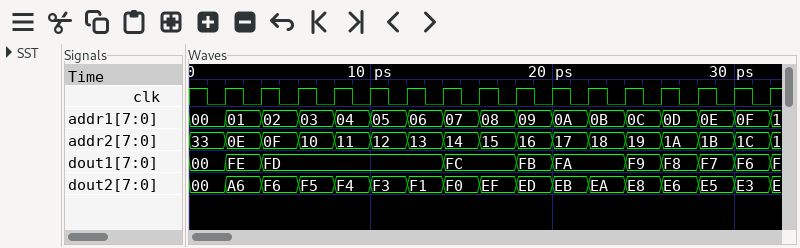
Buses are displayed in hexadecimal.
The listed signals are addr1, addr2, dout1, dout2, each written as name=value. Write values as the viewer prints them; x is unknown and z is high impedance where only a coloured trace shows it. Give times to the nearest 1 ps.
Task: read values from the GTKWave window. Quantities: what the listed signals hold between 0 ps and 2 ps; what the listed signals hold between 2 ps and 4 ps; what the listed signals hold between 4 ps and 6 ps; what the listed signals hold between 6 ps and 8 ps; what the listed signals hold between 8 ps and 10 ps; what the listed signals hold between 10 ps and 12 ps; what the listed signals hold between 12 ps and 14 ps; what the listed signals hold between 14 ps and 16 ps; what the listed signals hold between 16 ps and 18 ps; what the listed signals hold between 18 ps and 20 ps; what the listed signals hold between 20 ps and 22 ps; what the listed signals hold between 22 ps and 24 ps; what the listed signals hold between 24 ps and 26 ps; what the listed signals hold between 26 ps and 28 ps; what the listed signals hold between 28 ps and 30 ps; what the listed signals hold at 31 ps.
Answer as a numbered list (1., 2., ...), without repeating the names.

1. addr1=00, addr2=33, dout1=00, dout2=00
2. addr1=01, addr2=0E, dout1=FE, dout2=A6
3. addr1=02, addr2=0F, dout1=FD, dout2=F6
4. addr1=03, addr2=10, dout1=FD, dout2=F5
5. addr1=04, addr2=11, dout1=FD, dout2=F4
6. addr1=05, addr2=12, dout1=FD, dout2=F3
7. addr1=06, addr2=13, dout1=FD, dout2=F1
8. addr1=07, addr2=14, dout1=FC, dout2=F0
9. addr1=08, addr2=15, dout1=FC, dout2=EF
10. addr1=09, addr2=16, dout1=FB, dout2=ED
11. addr1=0A, addr2=17, dout1=FA, dout2=EB
12. addr1=0B, addr2=18, dout1=FA, dout2=EA
13. addr1=0C, addr2=19, dout1=F9, dout2=E8
14. addr1=0D, addr2=1A, dout1=F8, dout2=E6
15. addr1=0E, addr2=1B, dout1=F7, dout2=E5
16. addr1=0F, addr2=1C, dout1=F6, dout2=E3
